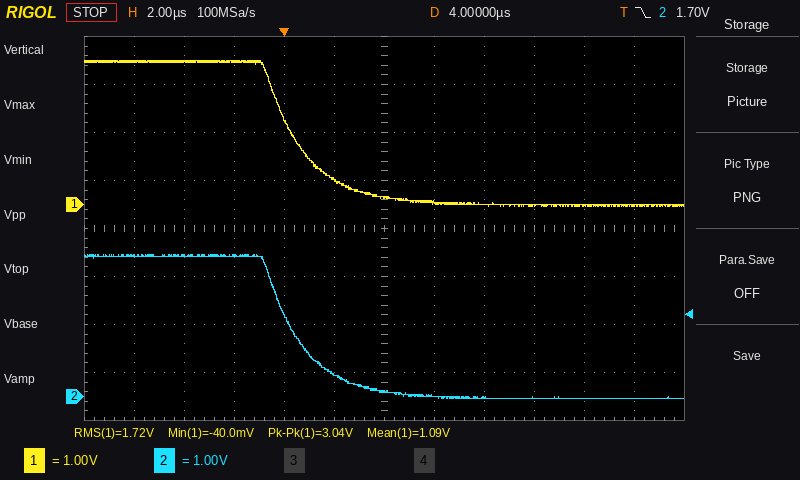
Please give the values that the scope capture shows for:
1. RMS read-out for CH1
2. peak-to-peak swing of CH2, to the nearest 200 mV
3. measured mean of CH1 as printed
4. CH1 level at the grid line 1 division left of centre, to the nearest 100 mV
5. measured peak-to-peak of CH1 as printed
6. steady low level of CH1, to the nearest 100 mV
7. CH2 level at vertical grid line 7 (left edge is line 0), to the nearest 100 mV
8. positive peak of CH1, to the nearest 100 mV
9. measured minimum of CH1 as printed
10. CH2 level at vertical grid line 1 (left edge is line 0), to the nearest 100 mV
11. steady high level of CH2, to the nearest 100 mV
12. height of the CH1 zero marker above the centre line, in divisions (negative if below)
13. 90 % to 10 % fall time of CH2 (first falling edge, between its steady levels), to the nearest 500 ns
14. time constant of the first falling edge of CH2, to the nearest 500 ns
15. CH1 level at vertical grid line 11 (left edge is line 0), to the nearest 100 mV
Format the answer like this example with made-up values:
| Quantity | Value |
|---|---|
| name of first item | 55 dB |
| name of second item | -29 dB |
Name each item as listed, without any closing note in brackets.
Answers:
| Quantity | Value |
|---|---|
| RMS read-out for CH1 | 1.72 V |
| peak-to-peak swing of CH2, to the nearest 200 mV | 3.0 V |
| measured mean of CH1 as printed | 1.09 V |
| CH1 level at the grid line 1 division left of centre, to the nearest 100 mV | 500 mV |
| measured peak-to-peak of CH1 as printed | 3.04 V |
| steady low level of CH1, to the nearest 100 mV | 0.0 V |
| CH2 level at vertical grid line 7 (left edge is line 0), to the nearest 100 mV | 0.0 V |
| positive peak of CH1, to the nearest 100 mV | 3.0 V |
| measured minimum of CH1 as printed | -40.0 mV |
| CH2 level at vertical grid line 1 (left edge is line 0), to the nearest 100 mV | 2.9 V |
| steady high level of CH2, to the nearest 100 mV | 2.9 V |
| height of the CH1 zero marker above the centre line, in divisions | +0.5 div |
| 90 % to 10 % fall time of CH2 (first falling edge, between its steady levels), to the nearest 500 ns | 3.5 µs |
| time constant of the first falling edge of CH2, to the nearest 500 ns | 1.5 µs |
| CH1 level at vertical grid line 11 (left edge is line 0), to the nearest 100 mV | 0.0 V |
